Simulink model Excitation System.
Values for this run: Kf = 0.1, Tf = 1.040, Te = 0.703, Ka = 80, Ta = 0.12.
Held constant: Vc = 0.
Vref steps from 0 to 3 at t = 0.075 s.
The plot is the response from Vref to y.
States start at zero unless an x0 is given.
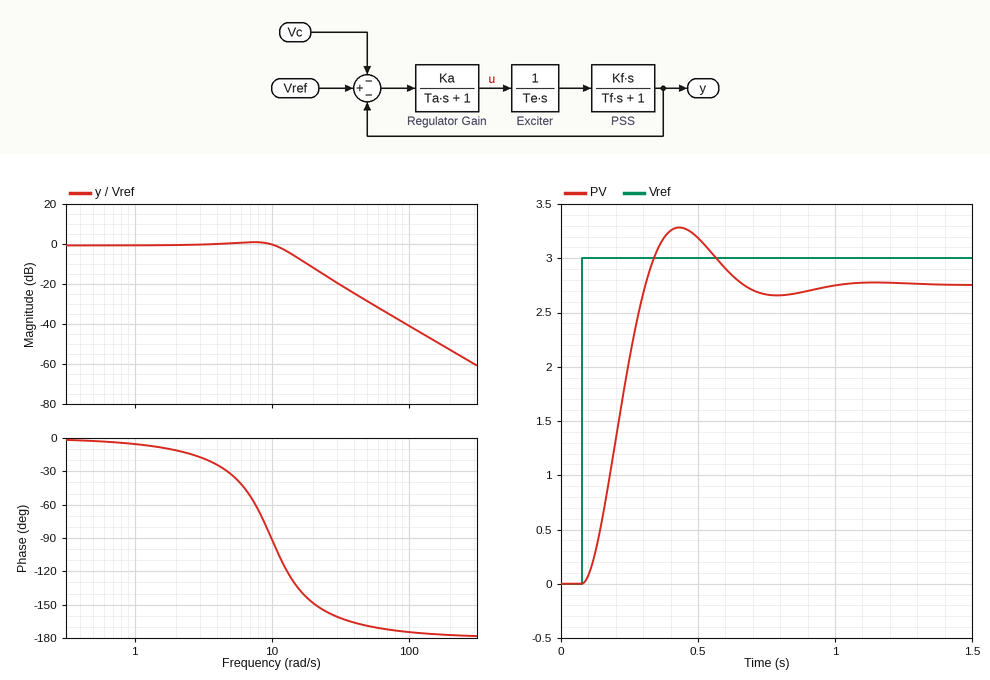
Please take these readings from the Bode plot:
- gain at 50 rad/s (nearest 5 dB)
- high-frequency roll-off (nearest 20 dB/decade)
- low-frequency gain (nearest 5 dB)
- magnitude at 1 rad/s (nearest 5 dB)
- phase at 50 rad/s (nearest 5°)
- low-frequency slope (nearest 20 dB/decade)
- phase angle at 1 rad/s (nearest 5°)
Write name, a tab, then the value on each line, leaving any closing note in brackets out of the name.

gain at 50 rad/s	-30 dB
high-frequency roll-off	-40 dB/decade
low-frequency gain	0 dB
magnitude at 1 rad/s	0 dB
phase at 50 rad/s	-170°
low-frequency slope	0 dB/decade
phase angle at 1 rad/s	-5°
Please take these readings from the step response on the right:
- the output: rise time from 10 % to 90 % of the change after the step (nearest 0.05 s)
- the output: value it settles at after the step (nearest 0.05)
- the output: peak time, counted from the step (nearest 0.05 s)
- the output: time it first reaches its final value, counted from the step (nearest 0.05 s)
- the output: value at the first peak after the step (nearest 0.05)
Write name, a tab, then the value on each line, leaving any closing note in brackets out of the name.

the output: rise time from 10 % to 90 % of the change after the step	0.15 s
the output: value it settles at after the step	2.75
the output: peak time, counted from the step	0.35 s
the output: time it first reaches its final value, counted from the step	0.25 s
the output: value at the first peak after the step	3.30
